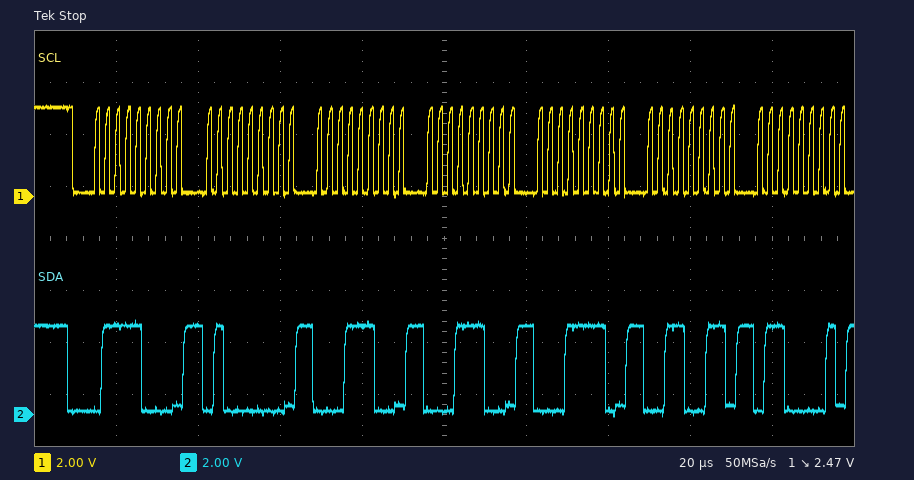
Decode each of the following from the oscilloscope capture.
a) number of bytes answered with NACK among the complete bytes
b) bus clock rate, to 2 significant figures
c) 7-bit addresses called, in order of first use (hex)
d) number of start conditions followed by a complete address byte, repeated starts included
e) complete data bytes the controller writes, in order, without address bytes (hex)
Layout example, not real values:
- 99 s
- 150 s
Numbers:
- 0
- 400 kHz
- 0x3C
- 1
- 40 1C 1C 1E 33 61
